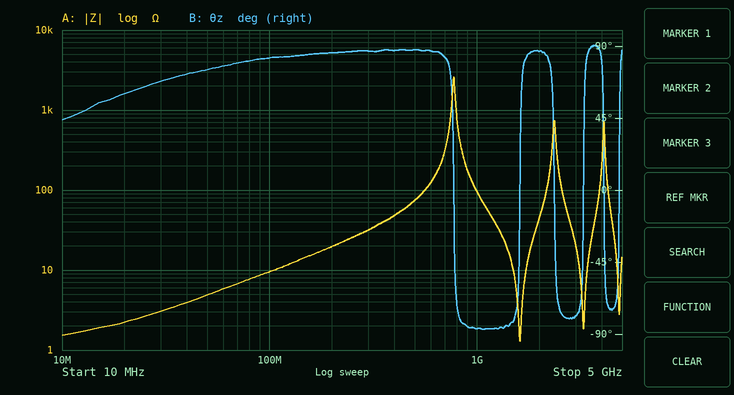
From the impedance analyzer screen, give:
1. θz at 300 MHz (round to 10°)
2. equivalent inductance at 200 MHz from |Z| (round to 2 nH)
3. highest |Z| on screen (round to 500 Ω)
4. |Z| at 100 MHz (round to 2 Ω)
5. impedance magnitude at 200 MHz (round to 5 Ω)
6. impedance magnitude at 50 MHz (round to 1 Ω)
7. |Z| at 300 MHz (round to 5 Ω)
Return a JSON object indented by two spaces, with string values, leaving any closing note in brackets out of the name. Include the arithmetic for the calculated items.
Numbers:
{
  "θz at 300 MHz": "90°",
  "equivalent inductance at 200 MHz from |Z|": "L = 20 Ω/(2π × 200 MHz) ≈ 16 nH",
  "highest |Z| on screen": "2.5 kΩ",
  "|Z| at 100 MHz": "10 Ω",
  "impedance magnitude at 200 MHz": "20 Ω",
  "impedance magnitude at 50 MHz": "5 Ω",
  "|Z| at 300 MHz": "30 Ω"
}
